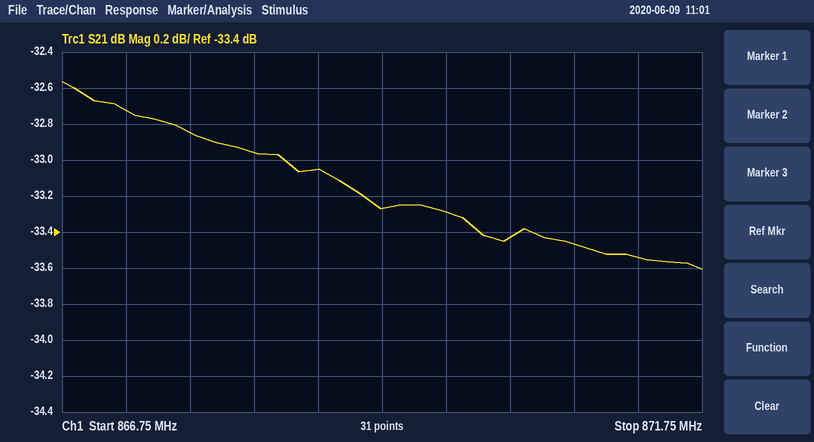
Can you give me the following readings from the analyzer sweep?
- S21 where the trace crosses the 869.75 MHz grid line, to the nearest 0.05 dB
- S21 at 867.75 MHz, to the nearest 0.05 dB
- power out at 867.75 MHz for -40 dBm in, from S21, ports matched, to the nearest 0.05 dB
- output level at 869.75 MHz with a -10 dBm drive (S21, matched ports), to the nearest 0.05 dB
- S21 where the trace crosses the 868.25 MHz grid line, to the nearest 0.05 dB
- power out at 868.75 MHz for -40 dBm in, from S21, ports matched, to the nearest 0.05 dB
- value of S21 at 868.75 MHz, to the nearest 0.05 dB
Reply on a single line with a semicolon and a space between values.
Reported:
-33.30 dB; -32.85 dB; -72.85 dBm; -43.30 dBm; -32.95 dB; -73.05 dBm; -33.05 dB
